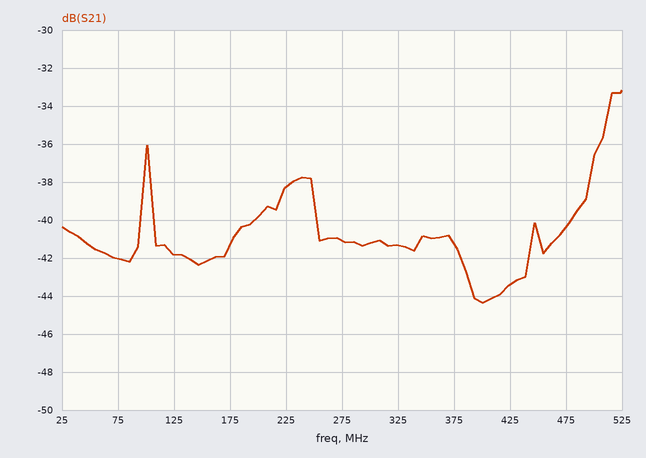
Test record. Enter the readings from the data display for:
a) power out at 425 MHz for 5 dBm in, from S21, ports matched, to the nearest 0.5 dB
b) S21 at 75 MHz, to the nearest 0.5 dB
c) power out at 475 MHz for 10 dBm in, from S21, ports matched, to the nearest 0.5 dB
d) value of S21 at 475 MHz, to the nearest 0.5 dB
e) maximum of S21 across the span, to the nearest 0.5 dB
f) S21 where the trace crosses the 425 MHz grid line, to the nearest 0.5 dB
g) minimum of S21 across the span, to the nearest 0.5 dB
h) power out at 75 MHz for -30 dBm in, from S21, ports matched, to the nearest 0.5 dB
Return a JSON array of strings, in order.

["-38.5 dBm", "-42.0 dB", "-30.5 dBm", "-40.5 dB", "-33.0 dB", "-43.5 dB", "-44.5 dB", "-72.0 dBm"]
